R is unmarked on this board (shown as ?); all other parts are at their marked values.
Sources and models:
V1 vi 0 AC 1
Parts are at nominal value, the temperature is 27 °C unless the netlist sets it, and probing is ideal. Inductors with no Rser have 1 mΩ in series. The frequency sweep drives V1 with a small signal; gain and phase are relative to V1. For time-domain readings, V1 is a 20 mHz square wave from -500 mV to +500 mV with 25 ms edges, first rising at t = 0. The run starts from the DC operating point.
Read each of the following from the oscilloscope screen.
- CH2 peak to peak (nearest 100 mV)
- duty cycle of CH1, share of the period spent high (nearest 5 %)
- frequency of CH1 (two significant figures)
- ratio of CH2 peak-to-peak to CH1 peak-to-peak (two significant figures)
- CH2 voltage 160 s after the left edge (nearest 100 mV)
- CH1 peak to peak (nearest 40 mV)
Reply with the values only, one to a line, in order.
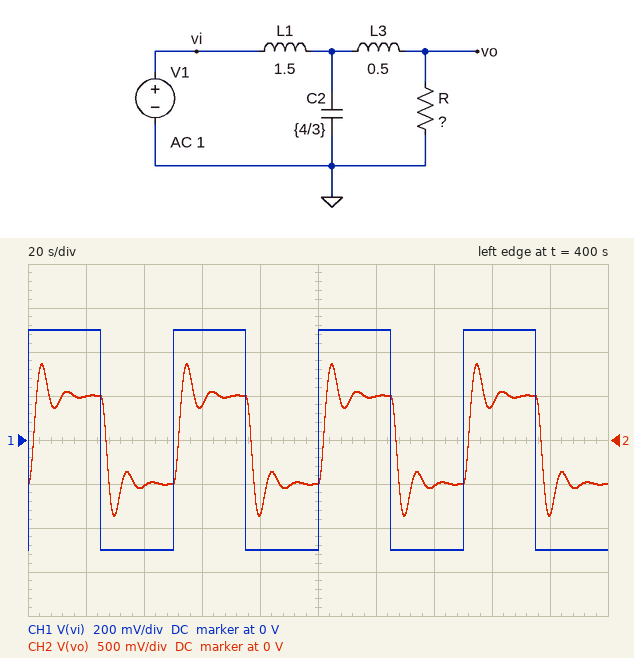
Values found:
1.7 V
50 %
20 mHz
1.7
400 mV
1.00 V
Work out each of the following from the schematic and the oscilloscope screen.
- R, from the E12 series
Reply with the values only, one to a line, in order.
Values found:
1.8 Ω
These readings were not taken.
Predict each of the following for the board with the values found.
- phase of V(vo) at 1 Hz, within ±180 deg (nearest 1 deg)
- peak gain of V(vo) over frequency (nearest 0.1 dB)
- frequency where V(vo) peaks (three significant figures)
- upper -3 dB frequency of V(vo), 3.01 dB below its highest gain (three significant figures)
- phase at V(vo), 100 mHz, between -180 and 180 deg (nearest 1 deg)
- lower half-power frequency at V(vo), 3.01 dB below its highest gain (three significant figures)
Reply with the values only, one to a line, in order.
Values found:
121 deg
4.6 dB
108 mHz
141 mHz
-69 deg
57.5 mHz
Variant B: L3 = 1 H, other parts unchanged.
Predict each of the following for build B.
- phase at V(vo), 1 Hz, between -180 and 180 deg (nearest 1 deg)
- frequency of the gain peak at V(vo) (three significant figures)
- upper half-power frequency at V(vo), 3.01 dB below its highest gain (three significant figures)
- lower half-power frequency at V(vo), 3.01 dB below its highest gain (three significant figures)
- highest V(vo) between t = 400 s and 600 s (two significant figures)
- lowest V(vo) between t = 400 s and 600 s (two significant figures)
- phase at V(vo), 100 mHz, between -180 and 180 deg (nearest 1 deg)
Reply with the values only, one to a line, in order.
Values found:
106 deg
117 mHz
148 mHz
65.0 mHz
850 mV
-850 mV
-71 deg
